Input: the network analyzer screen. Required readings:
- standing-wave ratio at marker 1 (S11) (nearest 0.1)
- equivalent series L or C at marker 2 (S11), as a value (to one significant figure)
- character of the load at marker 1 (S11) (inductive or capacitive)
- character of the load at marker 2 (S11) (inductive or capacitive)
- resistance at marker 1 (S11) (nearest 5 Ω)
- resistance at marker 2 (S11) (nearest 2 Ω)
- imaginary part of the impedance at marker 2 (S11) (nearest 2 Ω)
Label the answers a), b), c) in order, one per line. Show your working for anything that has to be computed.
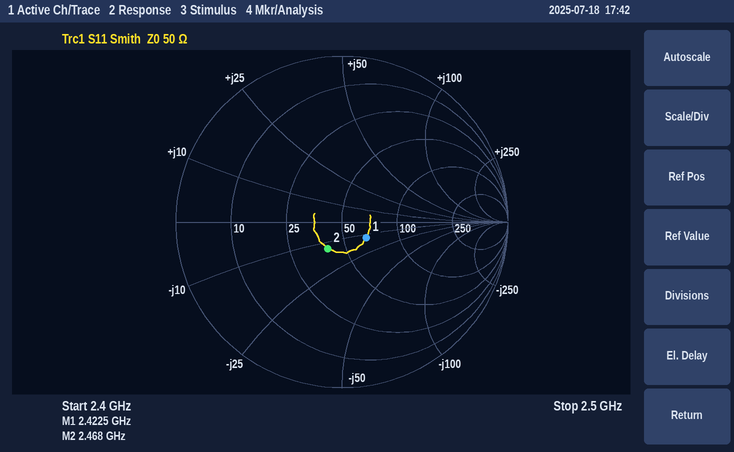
a) 1.4
b) C = 1/(2π × 2.468 GHz × 14 Ω) ≈ 5 pF
c) capacitive
d) capacitive
e) 65 Ω
f) 40 Ω
g) -14 Ω
